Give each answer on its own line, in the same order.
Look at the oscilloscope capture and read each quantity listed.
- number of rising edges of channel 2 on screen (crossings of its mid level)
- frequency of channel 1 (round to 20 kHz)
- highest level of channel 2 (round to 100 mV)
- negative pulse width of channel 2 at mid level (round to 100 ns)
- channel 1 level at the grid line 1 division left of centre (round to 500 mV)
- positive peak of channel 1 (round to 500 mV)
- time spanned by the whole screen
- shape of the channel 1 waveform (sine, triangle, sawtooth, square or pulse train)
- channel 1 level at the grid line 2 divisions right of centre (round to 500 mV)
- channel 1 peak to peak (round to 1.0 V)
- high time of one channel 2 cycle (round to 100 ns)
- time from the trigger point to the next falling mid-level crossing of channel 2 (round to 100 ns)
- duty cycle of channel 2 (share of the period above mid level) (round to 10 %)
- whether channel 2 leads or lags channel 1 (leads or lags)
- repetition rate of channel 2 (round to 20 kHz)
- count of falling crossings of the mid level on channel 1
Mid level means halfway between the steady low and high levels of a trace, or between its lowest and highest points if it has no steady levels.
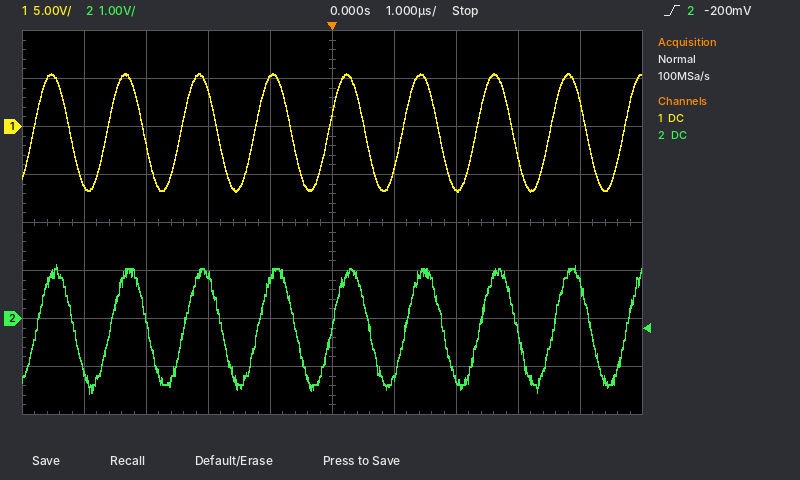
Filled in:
9
840 kHz
1.1 V
600 ns
5.0 V
5.5 V
10 µs
sine
-6.5 V
12.0 V
600 ns
600 ns
50 %
lags
840 kHz
8
